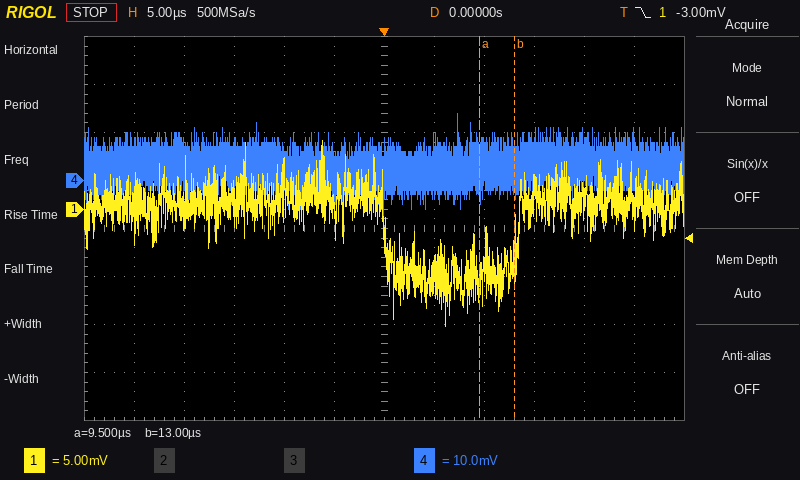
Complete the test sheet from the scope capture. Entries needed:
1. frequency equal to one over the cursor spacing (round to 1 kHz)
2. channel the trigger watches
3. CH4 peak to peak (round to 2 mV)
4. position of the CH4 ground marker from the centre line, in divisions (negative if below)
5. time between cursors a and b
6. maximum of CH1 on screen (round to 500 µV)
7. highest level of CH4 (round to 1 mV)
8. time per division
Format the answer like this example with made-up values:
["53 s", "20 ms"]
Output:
["286 kHz", "CH1", "22 mV", "+1.0 div", "3.5 µs", "7.0 mV", "14 mV", "5 µs"]
